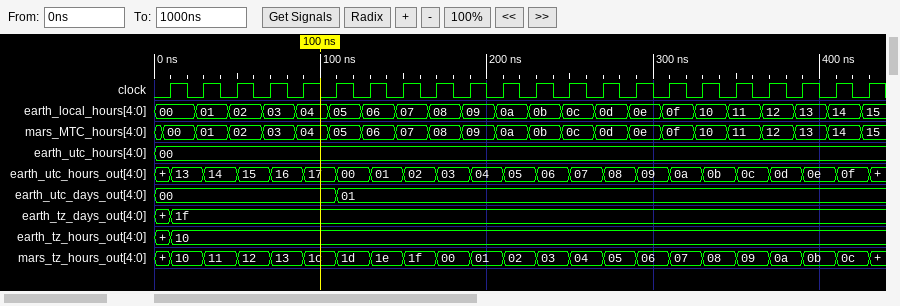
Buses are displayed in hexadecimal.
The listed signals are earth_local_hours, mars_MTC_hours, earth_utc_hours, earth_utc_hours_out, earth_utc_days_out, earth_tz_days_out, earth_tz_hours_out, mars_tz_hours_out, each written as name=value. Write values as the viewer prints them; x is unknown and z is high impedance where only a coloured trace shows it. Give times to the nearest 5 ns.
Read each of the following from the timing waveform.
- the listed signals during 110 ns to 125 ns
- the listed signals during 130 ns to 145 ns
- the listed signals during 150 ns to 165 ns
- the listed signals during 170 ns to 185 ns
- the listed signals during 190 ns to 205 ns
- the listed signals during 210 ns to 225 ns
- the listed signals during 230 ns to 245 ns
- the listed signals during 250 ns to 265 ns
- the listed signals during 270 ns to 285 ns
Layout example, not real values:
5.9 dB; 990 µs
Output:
earth_local_hours=05, mars_MTC_hours=05, earth_utc_hours=00, earth_utc_hours_out=00, earth_utc_days_out=01, earth_tz_days_out=1f, earth_tz_hours_out=10, mars_tz_hours_out=1d; earth_local_hours=06, mars_MTC_hours=06, earth_utc_hours=00, earth_utc_hours_out=01, earth_utc_days_out=01, earth_tz_days_out=1f, earth_tz_hours_out=10, mars_tz_hours_out=1e; earth_local_hours=07, mars_MTC_hours=07, earth_utc_hours=00, earth_utc_hours_out=02, earth_utc_days_out=01, earth_tz_days_out=1f, earth_tz_hours_out=10, mars_tz_hours_out=1f; earth_local_hours=08, mars_MTC_hours=08, earth_utc_hours=00, earth_utc_hours_out=03, earth_utc_days_out=01, earth_tz_days_out=1f, earth_tz_hours_out=10, mars_tz_hours_out=00; earth_local_hours=09, mars_MTC_hours=09, earth_utc_hours=00, earth_utc_hours_out=04, earth_utc_days_out=01, earth_tz_days_out=1f, earth_tz_hours_out=10, mars_tz_hours_out=01; earth_local_hours=0a, mars_MTC_hours=0a, earth_utc_hours=00, earth_utc_hours_out=05, earth_utc_days_out=01, earth_tz_days_out=1f, earth_tz_hours_out=10, mars_tz_hours_out=02; earth_local_hours=0b, mars_MTC_hours=0b, earth_utc_hours=00, earth_utc_hours_out=06, earth_utc_days_out=01, earth_tz_days_out=1f, earth_tz_hours_out=10, mars_tz_hours_out=03; earth_local_hours=0c, mars_MTC_hours=0c, earth_utc_hours=00, earth_utc_hours_out=07, earth_utc_days_out=01, earth_tz_days_out=1f, earth_tz_hours_out=10, mars_tz_hours_out=04; earth_local_hours=0d, mars_MTC_hours=0d, earth_utc_hours=00, earth_utc_hours_out=08, earth_utc_days_out=01, earth_tz_days_out=1f, earth_tz_hours_out=10, mars_tz_hours_out=05
